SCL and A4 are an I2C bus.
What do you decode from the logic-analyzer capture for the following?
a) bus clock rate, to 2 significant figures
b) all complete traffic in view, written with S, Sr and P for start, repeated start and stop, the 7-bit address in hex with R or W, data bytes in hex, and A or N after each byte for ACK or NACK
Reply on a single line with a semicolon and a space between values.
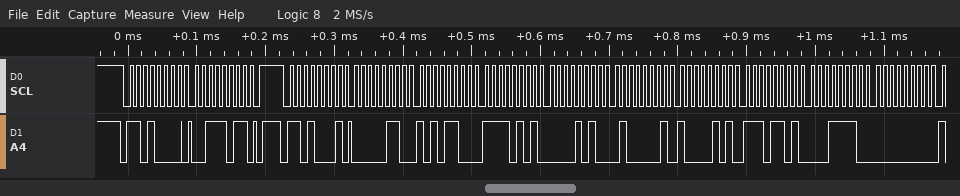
100 kHz; S 68W A 3B A P S 68R A 06 A AC A F5 A 0A A 41 A 85 A ED A 1E A 00 A
